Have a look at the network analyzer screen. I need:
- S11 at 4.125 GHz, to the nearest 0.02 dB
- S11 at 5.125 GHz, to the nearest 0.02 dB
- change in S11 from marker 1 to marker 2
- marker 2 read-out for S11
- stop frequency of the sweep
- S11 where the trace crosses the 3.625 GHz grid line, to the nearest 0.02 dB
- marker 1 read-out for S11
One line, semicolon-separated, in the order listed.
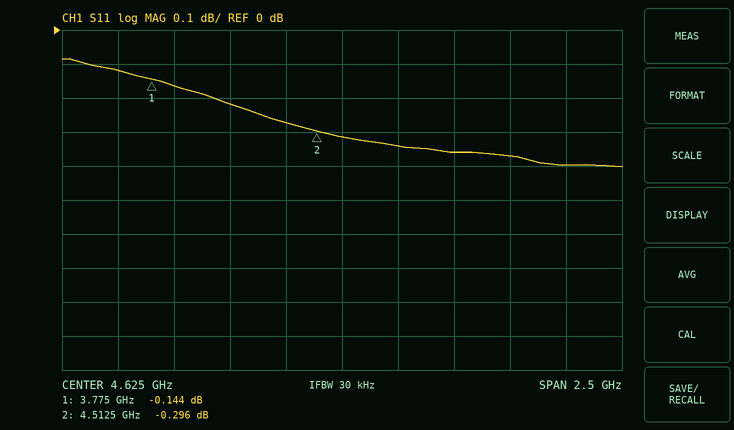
-0.22 dB; -0.36 dB; -0.152 dB; -0.296 dB; 5.875 GHz; -0.12 dB; -0.144 dB
